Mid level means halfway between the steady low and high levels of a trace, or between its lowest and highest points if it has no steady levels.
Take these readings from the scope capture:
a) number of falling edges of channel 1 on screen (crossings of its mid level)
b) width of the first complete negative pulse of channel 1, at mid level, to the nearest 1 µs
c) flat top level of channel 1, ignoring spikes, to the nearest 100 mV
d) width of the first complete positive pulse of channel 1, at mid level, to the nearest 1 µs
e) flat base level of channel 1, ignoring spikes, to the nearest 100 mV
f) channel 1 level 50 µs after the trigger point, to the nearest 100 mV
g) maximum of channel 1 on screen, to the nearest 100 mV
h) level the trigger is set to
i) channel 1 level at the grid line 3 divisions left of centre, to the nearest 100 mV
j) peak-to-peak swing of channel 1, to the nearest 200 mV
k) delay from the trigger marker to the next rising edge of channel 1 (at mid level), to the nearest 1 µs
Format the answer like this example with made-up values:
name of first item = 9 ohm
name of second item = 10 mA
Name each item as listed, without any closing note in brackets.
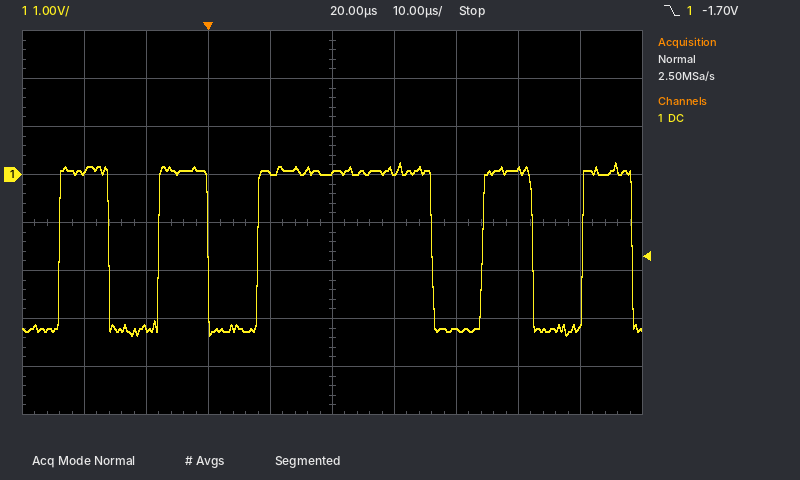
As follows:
number of falling edges of channel 1 on screen = 5
width of the first complete negative pulse of channel 1, at mid level, to the nearest 1 µs = 8 µs
flat top level of channel 1, ignoring spikes, to the nearest 100 mV = 100 mV
width of the first complete positive pulse of channel 1, at mid level, to the nearest 1 µs = 8 µs
flat base level of channel 1, ignoring spikes, to the nearest 100 mV = -3.2 V
channel 1 level 50 µs after the trigger point, to the nearest 100 mV = 100 mV
maximum of channel 1 on screen, to the nearest 100 mV = 200 mV
level the trigger is set to = -1.70 V
channel 1 level at the grid line 3 divisions left of centre, to the nearest 100 mV = -3.2 V
peak-to-peak swing of channel 1, to the nearest 200 mV = 3.6 V
delay from the trigger marker to the next rising edge of channel 1 (at mid level), to the nearest 1 µs = 8 µs
